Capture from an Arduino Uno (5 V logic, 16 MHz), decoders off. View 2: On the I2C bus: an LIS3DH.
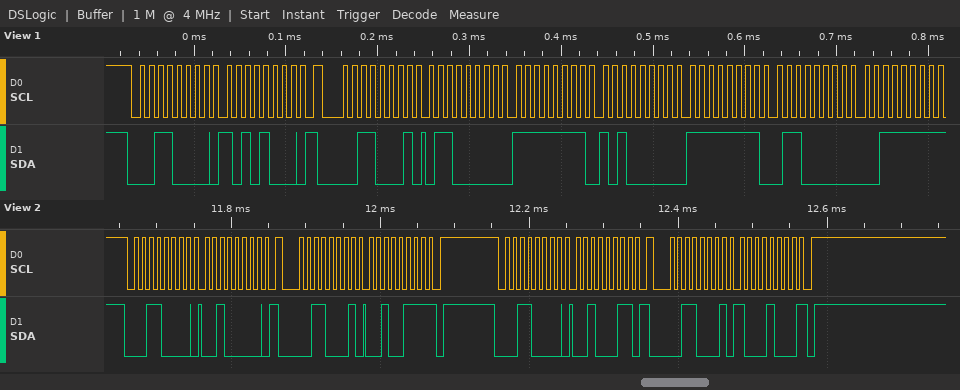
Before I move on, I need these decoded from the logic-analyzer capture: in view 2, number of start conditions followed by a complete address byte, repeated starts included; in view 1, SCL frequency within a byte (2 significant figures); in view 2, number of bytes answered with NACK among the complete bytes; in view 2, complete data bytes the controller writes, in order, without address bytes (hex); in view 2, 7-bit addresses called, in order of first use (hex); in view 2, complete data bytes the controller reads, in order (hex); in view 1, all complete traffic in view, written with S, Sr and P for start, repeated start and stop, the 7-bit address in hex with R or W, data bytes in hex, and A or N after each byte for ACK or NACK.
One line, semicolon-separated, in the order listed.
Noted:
4; 100 kHz; 2; 20 23; 0x18; 27 88; S 18W A A8 A Sr 18R A 60 A FF A A0 A FF A 60 A 3F N
